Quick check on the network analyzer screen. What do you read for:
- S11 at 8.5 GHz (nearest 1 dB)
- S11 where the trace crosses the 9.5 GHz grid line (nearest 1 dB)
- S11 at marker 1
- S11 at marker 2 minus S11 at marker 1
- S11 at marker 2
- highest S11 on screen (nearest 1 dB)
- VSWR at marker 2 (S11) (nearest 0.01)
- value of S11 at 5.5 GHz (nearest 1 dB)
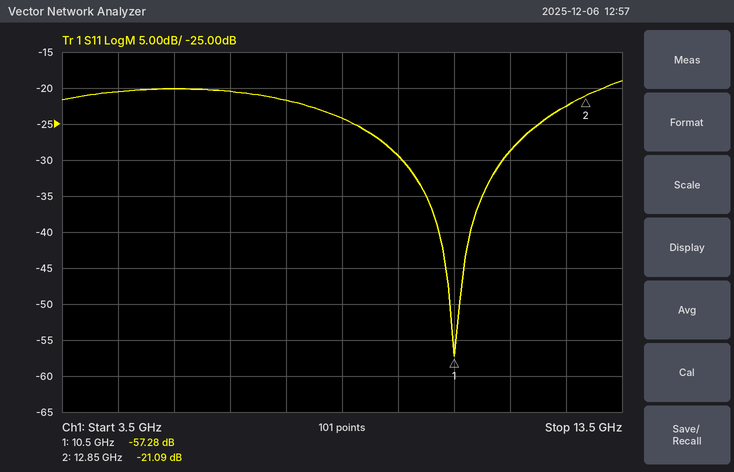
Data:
-24 dB
-29 dB
-57.28 dB
36.19 dB
-21.09 dB
-19 dB
1.19
-20 dB
